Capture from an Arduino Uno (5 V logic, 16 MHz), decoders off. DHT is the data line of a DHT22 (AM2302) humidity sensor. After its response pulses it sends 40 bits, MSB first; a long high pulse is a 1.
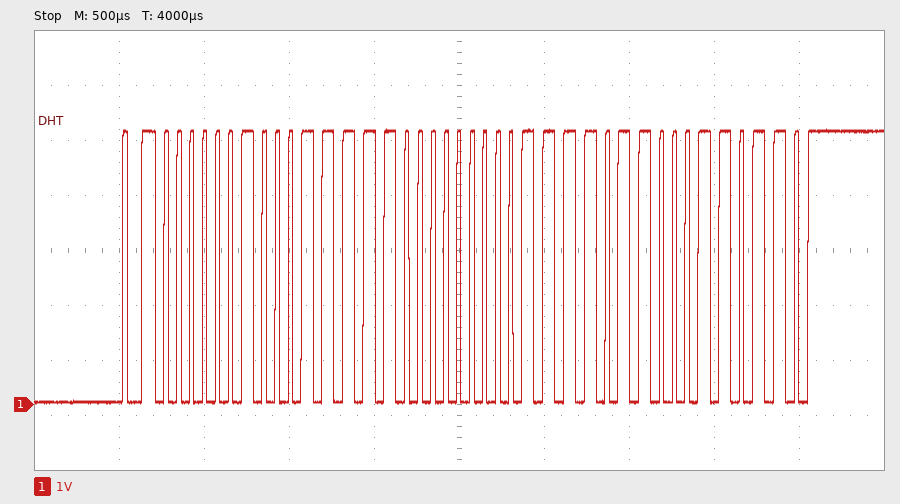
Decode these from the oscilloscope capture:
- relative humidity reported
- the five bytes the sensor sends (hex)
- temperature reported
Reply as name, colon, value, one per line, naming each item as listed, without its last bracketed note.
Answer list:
relative humidity reported: 57.4 %
the five bytes the sensor sends: 02 3E 00 F6 36
temperature reported: 24.6 °C
